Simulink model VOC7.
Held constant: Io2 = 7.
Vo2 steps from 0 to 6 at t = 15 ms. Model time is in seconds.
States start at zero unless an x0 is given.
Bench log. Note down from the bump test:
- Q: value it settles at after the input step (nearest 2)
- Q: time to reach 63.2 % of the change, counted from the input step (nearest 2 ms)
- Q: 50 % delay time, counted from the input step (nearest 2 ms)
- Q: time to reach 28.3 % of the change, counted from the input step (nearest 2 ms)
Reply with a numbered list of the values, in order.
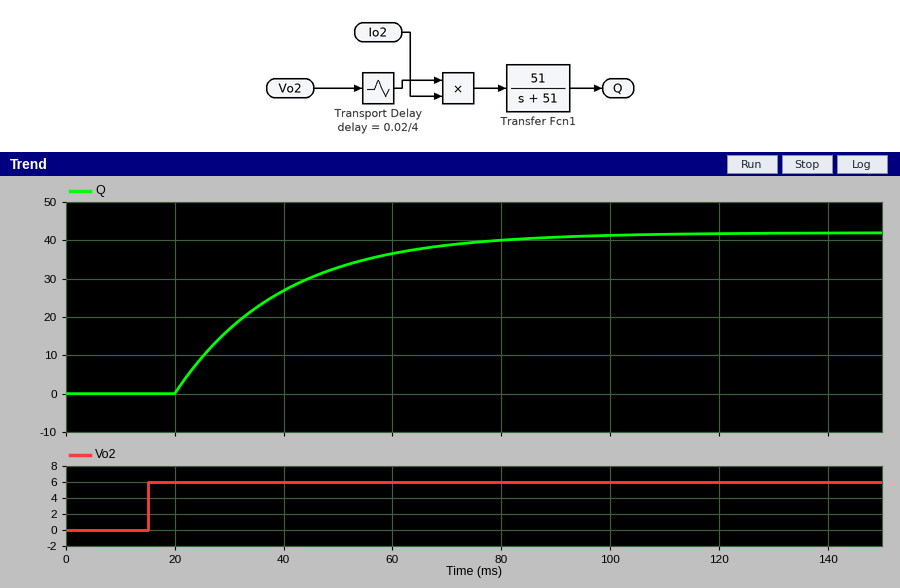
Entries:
1. 42
2. 24 ms
3. 18 ms
4. 12 ms
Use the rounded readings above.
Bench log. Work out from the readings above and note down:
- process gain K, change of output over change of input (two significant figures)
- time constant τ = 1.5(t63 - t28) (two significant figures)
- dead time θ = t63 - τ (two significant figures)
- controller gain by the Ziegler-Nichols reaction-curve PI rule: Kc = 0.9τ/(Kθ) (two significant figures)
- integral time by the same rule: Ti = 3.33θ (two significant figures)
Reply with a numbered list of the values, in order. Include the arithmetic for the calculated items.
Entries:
1. (42 - 0) / 6 = 7.0
2. 1.5 × (24 - 12) = 18 ms
3. 24 - 18 = 6.0 ms
4. 0.9 × 18 / (7 × 6) = 0.39
5. 3.33 × 6 = 20 ms
